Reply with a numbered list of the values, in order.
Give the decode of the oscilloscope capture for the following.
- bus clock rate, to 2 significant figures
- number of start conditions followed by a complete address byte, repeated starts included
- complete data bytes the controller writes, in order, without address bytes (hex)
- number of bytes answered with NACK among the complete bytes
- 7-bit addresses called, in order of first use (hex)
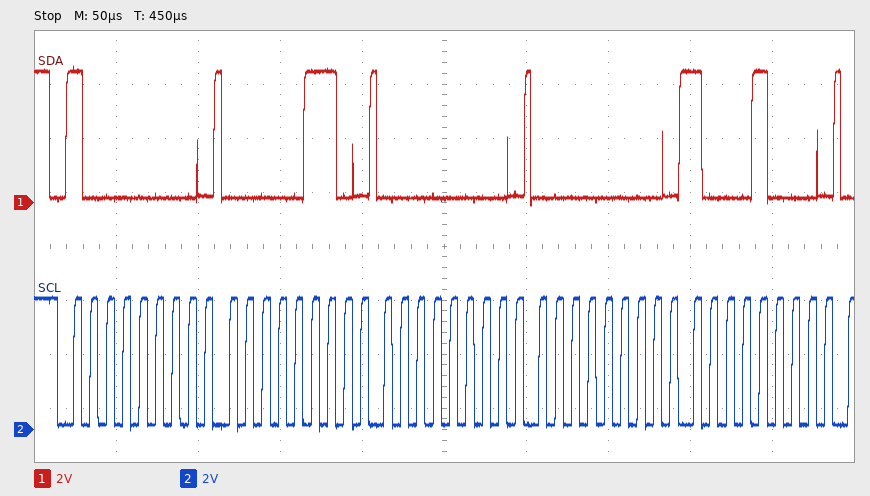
1. 100 kHz
2. 1
3. 06 00 00 88
4. 0
5. 0x40
